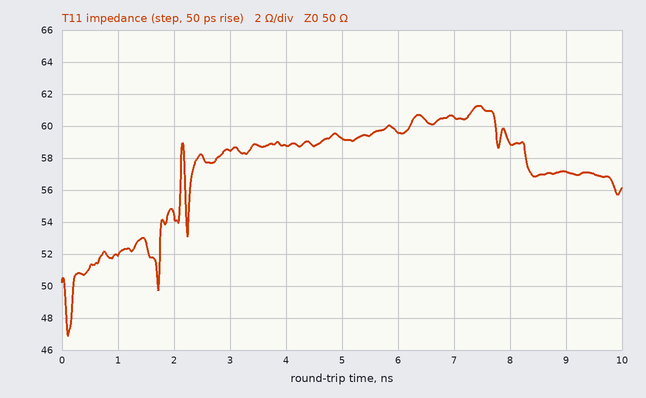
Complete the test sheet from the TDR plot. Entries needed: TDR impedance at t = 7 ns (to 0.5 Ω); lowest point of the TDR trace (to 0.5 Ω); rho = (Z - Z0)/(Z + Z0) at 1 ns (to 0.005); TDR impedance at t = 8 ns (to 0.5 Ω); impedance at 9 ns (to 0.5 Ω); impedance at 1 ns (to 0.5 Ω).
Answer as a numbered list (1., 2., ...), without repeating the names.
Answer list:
1. 60.5 Ω
2. 47.0 Ω
3. +0.020
4. 59.0 Ω
5. 57.0 Ω
6. 52.0 Ω
